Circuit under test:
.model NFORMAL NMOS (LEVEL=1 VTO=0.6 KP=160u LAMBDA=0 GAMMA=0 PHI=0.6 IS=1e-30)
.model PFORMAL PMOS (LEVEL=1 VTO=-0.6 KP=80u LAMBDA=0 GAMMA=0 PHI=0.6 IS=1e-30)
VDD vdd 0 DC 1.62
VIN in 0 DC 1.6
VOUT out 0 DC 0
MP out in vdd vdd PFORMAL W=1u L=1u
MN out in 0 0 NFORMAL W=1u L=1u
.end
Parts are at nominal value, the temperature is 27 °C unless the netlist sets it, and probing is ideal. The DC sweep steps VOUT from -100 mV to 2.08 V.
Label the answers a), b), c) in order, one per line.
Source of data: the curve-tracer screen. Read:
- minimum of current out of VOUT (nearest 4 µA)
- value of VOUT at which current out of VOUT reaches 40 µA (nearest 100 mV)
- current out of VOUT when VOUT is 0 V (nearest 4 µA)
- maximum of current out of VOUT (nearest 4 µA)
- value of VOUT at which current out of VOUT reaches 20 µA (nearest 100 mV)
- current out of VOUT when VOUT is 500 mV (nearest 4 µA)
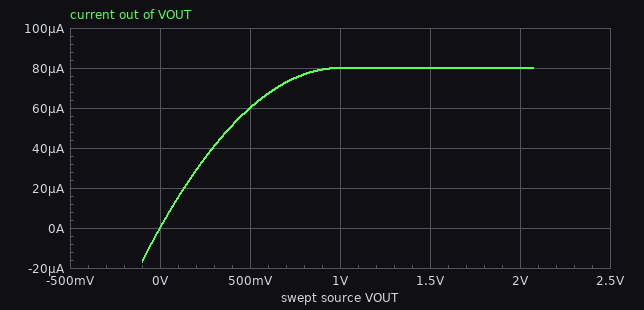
a) -16 µA
b) 300 mV
c) 0 A
d) 80 µA
e) 100 mV
f) 60 µA
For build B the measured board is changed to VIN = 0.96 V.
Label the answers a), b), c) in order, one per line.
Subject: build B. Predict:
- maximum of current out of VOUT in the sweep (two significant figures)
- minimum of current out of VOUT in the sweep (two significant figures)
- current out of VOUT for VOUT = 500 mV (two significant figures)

a) 21 µA
b) -6.7 µA
c) 10 µA
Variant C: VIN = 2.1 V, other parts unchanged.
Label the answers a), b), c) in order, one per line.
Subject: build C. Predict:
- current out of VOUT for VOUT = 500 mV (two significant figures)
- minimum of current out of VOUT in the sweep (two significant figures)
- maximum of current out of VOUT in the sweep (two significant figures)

a) 100 µA
b) -25 µA
c) 180 µA
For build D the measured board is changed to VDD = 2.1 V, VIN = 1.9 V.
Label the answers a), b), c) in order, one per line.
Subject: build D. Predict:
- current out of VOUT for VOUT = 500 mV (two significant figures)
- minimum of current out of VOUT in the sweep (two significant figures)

a) 84 µA
b) -22 µA
